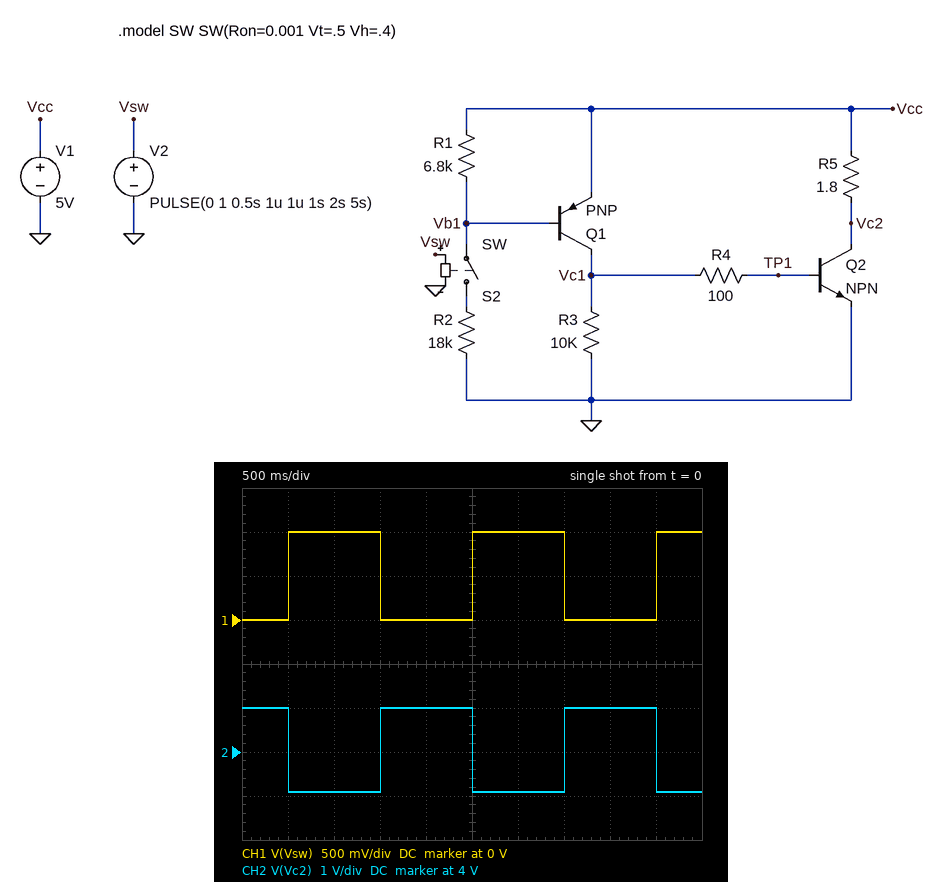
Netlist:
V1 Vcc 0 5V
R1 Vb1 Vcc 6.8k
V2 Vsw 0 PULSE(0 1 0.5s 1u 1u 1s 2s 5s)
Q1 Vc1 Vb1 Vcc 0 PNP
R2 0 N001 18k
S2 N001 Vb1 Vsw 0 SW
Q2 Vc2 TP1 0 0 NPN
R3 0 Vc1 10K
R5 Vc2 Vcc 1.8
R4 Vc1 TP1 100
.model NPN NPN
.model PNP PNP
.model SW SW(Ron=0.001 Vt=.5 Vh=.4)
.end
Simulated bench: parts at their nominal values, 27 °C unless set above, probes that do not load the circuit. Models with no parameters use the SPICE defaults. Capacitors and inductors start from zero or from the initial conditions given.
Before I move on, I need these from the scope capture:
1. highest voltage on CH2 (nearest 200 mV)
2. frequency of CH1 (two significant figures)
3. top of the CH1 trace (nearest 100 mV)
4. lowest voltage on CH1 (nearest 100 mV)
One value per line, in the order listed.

5.0 V
500 mHz
1.0 V
0 V
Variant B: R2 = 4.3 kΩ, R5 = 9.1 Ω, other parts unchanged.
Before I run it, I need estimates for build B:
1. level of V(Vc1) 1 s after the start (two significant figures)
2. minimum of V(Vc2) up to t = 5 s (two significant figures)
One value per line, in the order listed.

4.9 V
75 mV
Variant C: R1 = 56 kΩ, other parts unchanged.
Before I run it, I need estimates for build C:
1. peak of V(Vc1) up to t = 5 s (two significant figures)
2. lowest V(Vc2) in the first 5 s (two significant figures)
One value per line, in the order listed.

3.1 V
1.2 V
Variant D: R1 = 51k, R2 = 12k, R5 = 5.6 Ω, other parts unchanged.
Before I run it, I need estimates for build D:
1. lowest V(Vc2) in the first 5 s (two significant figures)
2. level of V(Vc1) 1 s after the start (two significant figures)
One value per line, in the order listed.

95 mV
4.2 V
